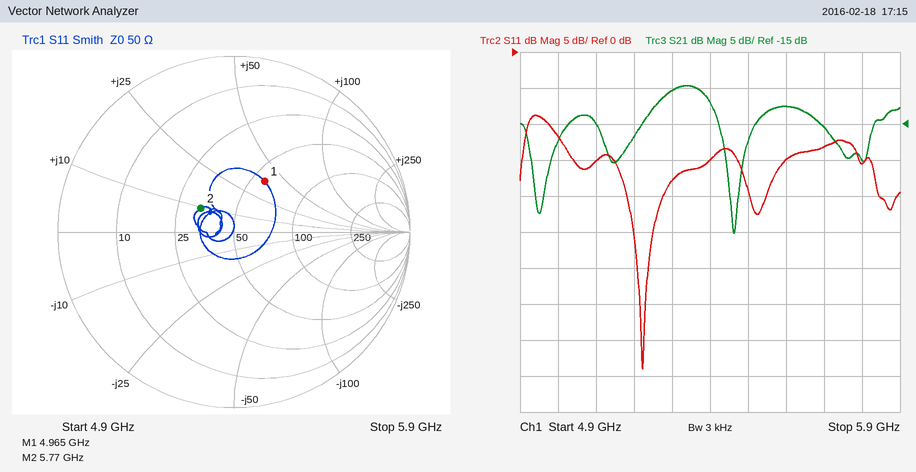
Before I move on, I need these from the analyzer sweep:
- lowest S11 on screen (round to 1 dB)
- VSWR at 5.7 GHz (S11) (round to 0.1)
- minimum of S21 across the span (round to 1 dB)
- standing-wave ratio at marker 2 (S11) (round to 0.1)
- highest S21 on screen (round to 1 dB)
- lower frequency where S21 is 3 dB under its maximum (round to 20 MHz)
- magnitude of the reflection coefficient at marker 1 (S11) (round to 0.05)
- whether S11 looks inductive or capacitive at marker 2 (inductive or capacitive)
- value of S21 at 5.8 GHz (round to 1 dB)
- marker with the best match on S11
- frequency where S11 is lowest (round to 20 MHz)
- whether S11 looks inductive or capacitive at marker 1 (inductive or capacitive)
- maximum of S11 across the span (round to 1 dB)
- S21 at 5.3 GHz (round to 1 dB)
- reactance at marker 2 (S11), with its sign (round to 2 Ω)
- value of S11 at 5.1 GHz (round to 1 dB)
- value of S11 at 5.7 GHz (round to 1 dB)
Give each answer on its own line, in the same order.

-44 dB
1.6
-30 dB
1.6
-10 dB
5.26 GHz
0.35
inductive
-20 dB
marker 2
5.22 GHz
inductive
-9 dB
-10 dB
+10 Ω
-15 dB
-13 dB
